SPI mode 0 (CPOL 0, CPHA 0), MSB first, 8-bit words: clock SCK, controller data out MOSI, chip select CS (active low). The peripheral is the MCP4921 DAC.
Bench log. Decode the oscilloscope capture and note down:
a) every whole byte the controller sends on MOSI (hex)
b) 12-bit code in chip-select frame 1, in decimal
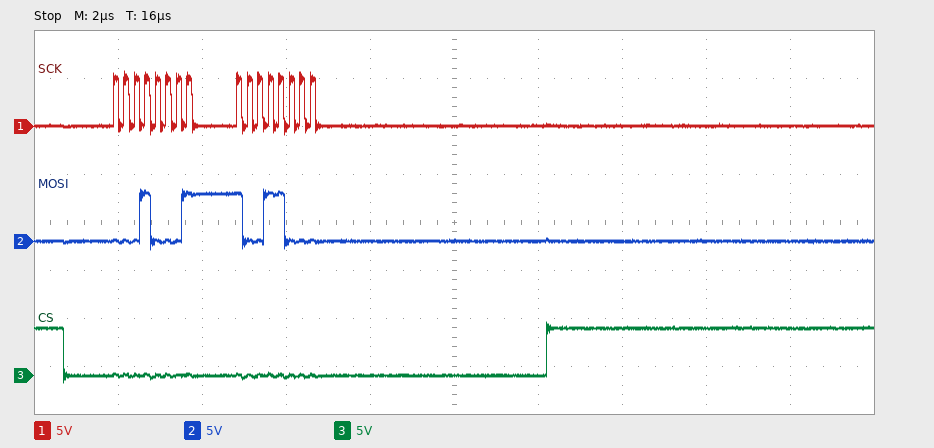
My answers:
11 98
408
